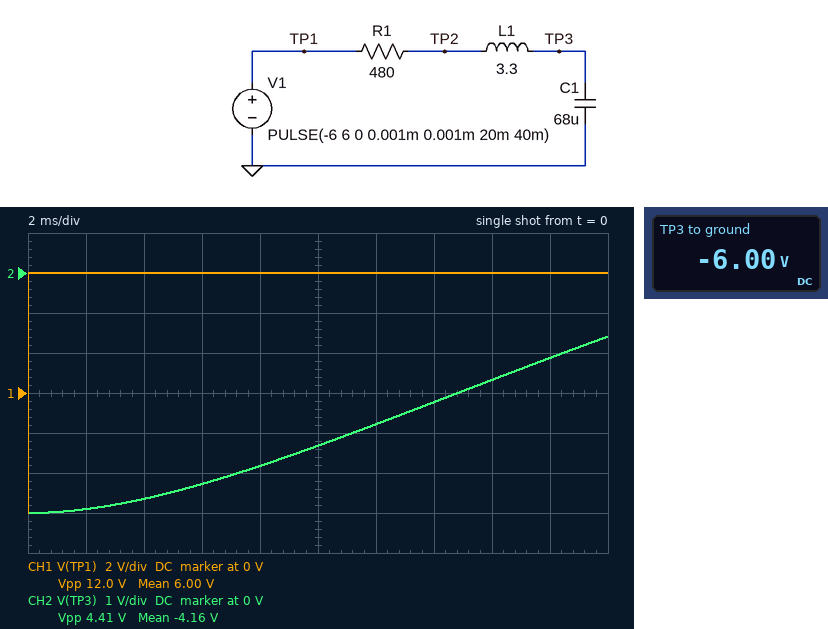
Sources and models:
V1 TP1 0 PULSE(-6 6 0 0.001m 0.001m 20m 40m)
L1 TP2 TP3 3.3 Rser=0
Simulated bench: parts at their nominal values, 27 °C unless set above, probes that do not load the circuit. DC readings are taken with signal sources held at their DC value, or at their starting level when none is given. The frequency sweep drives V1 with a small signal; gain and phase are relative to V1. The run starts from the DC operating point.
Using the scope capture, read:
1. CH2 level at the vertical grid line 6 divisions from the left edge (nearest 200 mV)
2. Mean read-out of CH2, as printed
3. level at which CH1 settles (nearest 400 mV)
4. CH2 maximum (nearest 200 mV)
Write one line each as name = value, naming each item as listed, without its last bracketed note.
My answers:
CH2 level at the vertical grid line 6 divisions from the left edge = -3.8 V
Mean read-out of CH2, as printed = -4.16 V
level at which CH1 settles = 6.0 V
CH2 maximum = -1.6 V
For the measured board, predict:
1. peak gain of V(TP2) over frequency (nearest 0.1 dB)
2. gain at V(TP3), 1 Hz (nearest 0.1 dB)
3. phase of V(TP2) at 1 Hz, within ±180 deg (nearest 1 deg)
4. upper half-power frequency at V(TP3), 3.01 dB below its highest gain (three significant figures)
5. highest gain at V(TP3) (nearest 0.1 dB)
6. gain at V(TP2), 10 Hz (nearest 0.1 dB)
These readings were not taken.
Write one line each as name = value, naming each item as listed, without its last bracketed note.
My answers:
peak gain of V(TP2) over frequency = 0 dB
gain at V(TP3), 1 Hz = -0.1 dB
phase of V(TP2) at 1 Hz, within ±180 deg = -12 deg
upper half-power frequency at V(TP3), 3.01 dB below its highest gain = 6.06 Hz
highest gain at V(TP3) = 0 dB
gain at V(TP2), 10 Hz = -25.1 dB
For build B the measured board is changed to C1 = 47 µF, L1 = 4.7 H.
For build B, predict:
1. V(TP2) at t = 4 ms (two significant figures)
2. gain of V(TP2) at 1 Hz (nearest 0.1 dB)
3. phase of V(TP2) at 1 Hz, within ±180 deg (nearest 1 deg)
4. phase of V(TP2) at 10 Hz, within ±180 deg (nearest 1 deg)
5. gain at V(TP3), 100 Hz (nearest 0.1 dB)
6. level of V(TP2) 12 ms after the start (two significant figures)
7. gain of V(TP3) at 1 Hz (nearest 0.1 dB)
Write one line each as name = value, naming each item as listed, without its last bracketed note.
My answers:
V(TP2) at t = 4 ms = 2.0 V
gain of V(TP2) at 1 Hz = -0.1 dB
phase of V(TP2) at 1 Hz, within ±180 deg = -8 deg
phase of V(TP2) at 10 Hz, within ±180 deg = -85 deg
gain at V(TP3), 100 Hz = -38.8 dB
level of V(TP2) 12 ms after the start = -1.6 V
gain of V(TP3) at 1 Hz = 0 dB
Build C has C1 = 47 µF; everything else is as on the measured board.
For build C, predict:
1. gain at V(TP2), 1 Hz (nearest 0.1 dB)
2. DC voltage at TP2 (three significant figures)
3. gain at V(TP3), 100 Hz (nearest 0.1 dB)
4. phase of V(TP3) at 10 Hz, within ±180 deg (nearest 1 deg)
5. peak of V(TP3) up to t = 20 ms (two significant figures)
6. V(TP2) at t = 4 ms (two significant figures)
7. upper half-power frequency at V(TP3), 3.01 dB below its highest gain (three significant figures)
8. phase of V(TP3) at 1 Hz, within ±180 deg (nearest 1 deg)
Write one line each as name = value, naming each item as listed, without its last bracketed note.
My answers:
gain at V(TP2), 1 Hz = -0.1 dB
DC voltage at TP2 = -6.00 V
gain at V(TP3), 100 Hz = -35.8 dB
phase of V(TP3) at 10 Hz, within ±180 deg = -75 deg
peak of V(TP3) up to t = 20 ms = 55 mV
V(TP2) at t = 4 ms = 800 mV
upper half-power frequency at V(TP3), 3.01 dB below its highest gain = 9.45 Hz
phase of V(TP3) at 1 Hz, within ±180 deg = -8 deg
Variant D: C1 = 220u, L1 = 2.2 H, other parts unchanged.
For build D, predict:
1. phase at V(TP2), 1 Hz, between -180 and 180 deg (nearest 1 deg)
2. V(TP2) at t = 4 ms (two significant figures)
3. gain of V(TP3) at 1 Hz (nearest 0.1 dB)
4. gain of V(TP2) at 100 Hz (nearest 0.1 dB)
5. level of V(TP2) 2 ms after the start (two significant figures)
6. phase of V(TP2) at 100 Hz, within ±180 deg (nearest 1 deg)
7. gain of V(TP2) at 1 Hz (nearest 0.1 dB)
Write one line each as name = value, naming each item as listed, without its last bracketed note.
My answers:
phase at V(TP2), 1 Hz, between -180 and 180 deg = -34 deg
V(TP2) at t = 4 ms = -950 mV
gain of V(TP3) at 1 Hz = -1.5 dB
gain of V(TP2) at 100 Hz = -0.5 dB
level of V(TP2) 2 ms after the start = 1.8 V
phase of V(TP2) at 100 Hz, within ±180 deg = 19 deg
gain of V(TP2) at 1 Hz = -1.6 dB
